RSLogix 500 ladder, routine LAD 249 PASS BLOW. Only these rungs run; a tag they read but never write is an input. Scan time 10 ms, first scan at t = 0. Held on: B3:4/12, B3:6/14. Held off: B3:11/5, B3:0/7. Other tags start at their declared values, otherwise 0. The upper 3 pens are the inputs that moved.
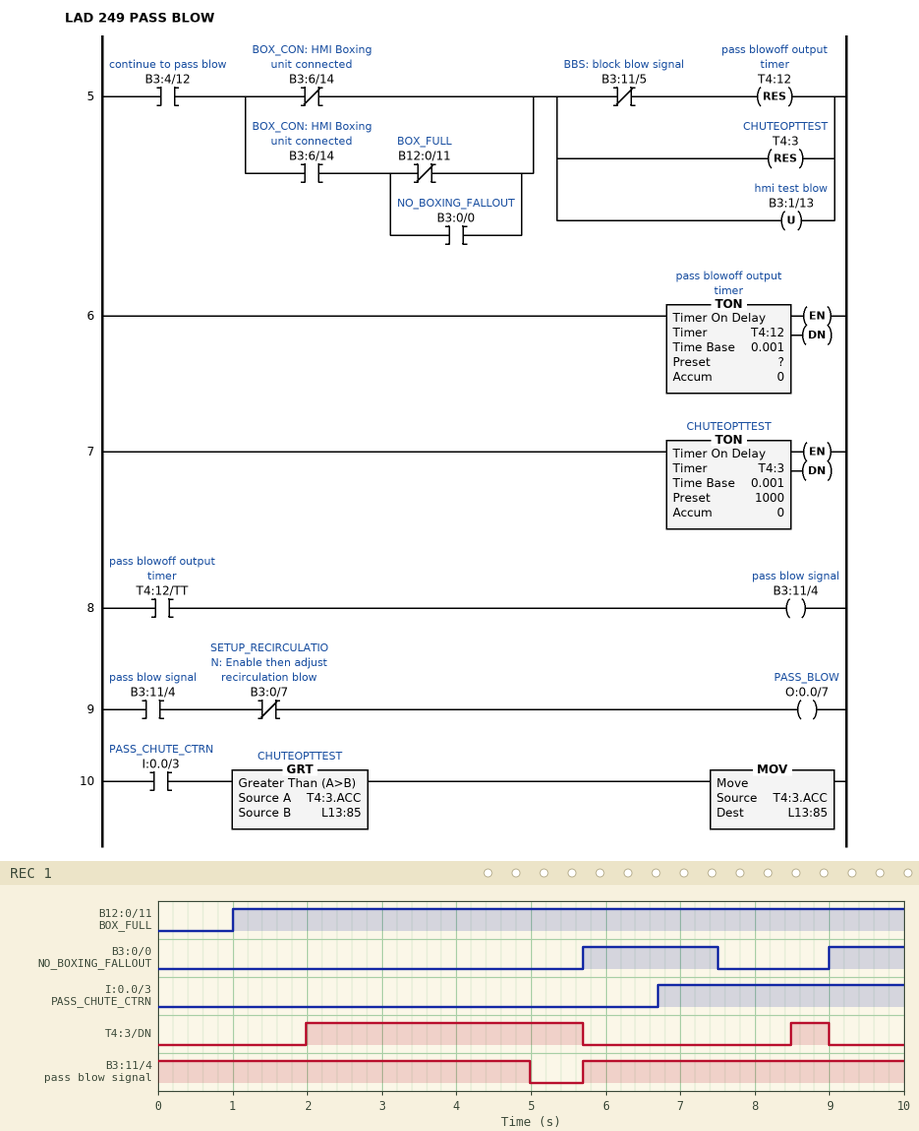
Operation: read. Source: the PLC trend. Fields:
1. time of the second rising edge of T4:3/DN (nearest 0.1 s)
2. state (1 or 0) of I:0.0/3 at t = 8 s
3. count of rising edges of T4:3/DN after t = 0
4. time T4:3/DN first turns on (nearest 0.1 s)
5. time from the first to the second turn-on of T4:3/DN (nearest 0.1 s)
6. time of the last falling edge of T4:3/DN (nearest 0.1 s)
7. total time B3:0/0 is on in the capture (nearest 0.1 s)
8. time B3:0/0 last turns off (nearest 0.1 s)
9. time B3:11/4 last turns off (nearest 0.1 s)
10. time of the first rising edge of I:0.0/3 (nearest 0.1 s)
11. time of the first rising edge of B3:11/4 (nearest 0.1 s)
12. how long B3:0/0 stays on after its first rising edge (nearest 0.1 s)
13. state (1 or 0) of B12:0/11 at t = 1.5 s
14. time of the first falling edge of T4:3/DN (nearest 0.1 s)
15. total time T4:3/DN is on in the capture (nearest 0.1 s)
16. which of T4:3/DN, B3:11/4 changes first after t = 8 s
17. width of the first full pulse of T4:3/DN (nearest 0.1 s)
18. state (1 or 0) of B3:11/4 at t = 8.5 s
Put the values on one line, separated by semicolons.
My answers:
8.5 s; 1; 2; 2.0 s; 6.5 s; 9.0 s; 2.8 s; 7.5 s; 5.0 s; 6.7 s; 5.7 s; 1.8 s; 1; 5.7 s; 4.2 s; T4:3/DN; 3.7 s; 1
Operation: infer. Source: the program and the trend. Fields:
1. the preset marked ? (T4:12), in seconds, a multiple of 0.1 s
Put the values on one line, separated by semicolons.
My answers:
4.0 s
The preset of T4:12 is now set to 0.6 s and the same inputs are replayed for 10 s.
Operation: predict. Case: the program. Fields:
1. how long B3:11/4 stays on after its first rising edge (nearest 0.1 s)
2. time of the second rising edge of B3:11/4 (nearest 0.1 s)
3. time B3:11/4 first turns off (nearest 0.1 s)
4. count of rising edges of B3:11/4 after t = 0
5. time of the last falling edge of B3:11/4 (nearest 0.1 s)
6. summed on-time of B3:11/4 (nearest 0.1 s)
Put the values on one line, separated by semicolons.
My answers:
2.4 s; 9.0 s; 1.6 s; 2; 8.1 s; 5.0 s
